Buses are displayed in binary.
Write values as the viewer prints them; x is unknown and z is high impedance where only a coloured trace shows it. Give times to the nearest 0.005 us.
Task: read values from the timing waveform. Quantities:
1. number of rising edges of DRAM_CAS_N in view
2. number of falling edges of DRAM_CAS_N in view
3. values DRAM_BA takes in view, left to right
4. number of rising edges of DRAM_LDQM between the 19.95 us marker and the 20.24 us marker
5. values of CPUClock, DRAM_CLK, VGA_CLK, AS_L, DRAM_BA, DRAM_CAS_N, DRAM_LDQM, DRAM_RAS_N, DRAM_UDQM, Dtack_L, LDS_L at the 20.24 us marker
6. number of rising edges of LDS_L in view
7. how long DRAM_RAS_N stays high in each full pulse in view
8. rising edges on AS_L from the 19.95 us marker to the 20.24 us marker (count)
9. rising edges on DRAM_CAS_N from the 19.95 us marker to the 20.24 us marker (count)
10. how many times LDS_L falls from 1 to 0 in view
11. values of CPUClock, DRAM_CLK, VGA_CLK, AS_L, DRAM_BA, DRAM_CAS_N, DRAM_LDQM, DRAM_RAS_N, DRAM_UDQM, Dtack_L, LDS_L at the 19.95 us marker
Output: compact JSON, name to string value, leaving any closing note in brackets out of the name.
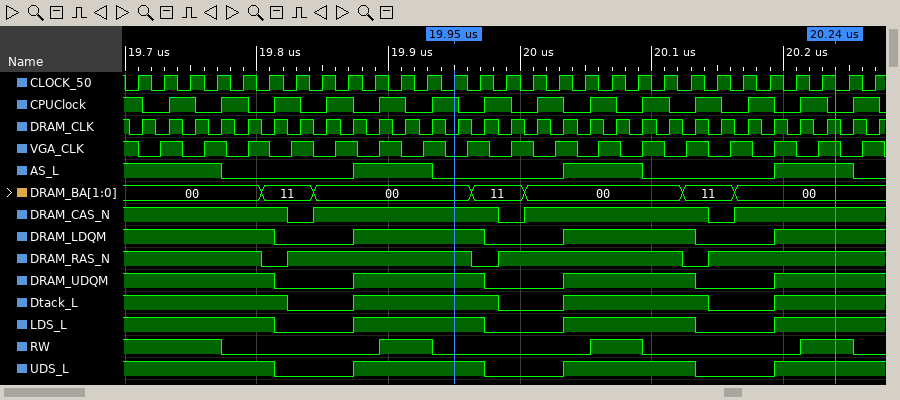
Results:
{"number of rising edges of DRAM_CAS_N in view": "3", "number of falling edges of DRAM_CAS_N in view": "3", "values DRAM_BA takes in view, left to right": "00, 11, 00, 11, 00, 11, 00", "number of rising edges of DRAM_LDQM between the 19.95 us marker and the 20.24 us marker": "2", "values of CPUClock, DRAM_CLK, VGA_CLK, AS_L, DRAM_BA, DRAM_CAS_N, DRAM_LDQM, DRAM_RAS_N, DRAM_UDQM, Dtack_L, LDS_L at the 20.24 us marker": "CPUClock=0, DRAM_CLK=1, VGA_CLK=1, AS_L=1, DRAM_BA=00, DRAM_CAS_N=1, DRAM_LDQM=1, DRAM_RAS_N=1, DRAM_UDQM=1, Dtack_L=1, LDS_L=1", "number of rising edges of LDS_L in view": "3", "how long DRAM_RAS_N stays high in each full pulse in view": "0.14 us, 0.14 us", "rising edges on AS_L from the 19.95 us marker to the 20.24 us marker": "2", "rising edges on DRAM_CAS_N from the 19.95 us marker to the 20.24 us marker": "2", "how many times LDS_L falls from 1 to 0 in view": "3", "values of CPUClock, DRAM_CLK, VGA_CLK, AS_L, DRAM_BA, DRAM_CAS_N, DRAM_LDQM, DRAM_RAS_N, DRAM_UDQM, Dtack_L, LDS_L at the 19.95 us marker": "CPUClock=1, DRAM_CLK=0, VGA_CLK=0, AS_L=0, DRAM_BA=00, DRAM_CAS_N=1, DRAM_LDQM=1, DRAM_RAS_N=1, DRAM_UDQM=1, Dtack_L=1, LDS_L=1"}
